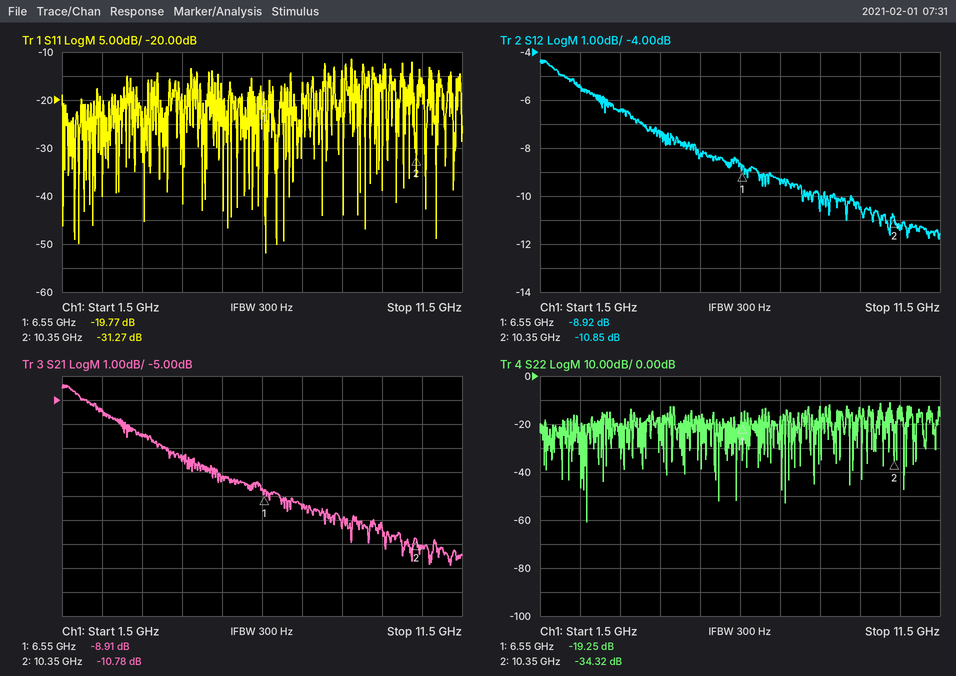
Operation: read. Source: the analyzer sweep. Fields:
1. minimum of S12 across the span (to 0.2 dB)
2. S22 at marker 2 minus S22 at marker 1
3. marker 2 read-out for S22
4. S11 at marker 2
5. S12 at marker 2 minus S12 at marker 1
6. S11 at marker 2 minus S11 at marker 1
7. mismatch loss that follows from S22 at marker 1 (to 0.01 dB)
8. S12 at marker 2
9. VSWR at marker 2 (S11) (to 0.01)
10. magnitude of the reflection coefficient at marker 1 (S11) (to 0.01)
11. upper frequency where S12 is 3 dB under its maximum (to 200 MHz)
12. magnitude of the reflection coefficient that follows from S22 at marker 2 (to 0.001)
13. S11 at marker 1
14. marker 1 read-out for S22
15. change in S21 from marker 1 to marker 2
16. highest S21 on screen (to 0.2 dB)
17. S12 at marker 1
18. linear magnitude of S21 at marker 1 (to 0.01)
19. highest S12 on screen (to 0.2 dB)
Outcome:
-11.8 dB
-15.07 dB
-34.32 dB
-31.27 dB
-1.93 dB
-11.50 dB
0.05 dB
-10.85 dB
1.06
0.10
4.4 GHz
0.019
-19.77 dB
-19.25 dB
-1.87 dB
-4.4 dB
-8.92 dB
0.36
-4.4 dB
